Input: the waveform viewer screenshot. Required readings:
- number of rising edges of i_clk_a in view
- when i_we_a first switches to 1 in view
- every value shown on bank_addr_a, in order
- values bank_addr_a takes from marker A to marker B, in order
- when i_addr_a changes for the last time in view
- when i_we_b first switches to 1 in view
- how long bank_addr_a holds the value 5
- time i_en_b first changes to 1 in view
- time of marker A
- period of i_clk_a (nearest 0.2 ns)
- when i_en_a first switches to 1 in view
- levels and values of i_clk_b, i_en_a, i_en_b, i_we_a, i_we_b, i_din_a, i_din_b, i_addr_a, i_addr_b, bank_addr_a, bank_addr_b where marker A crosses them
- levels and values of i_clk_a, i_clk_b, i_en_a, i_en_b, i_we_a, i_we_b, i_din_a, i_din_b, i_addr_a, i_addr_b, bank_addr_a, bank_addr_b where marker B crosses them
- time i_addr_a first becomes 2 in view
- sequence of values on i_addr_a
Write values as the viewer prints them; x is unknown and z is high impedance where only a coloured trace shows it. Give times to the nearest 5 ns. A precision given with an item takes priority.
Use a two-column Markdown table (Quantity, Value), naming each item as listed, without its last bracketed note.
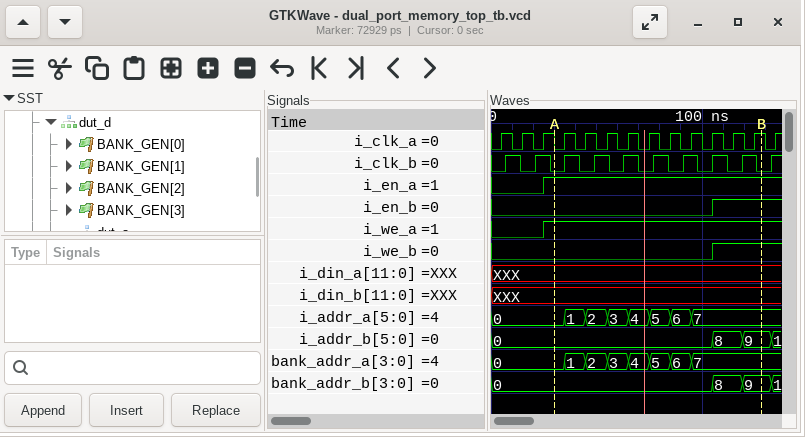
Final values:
| Quantity | Value |
|---|---|
| number of rising edges of i_clk_a in view | 14 |
| when i_we_a first switches to 1 in view | 25 ns |
| every value shown on bank_addr_a, in order | 0, 1, 2, 3, 4, 5, 6, 7 |
| values bank_addr_a takes from marker A to marker B, in order | 0, 1, 2, 3, 4, 5, 6, 7 |
| when i_addr_a changes for the last time in view | 95 ns |
| when i_we_b first switches to 1 in view | 105 ns |
| how long bank_addr_a holds the value 5 | 10 ns |
| time i_en_b first changes to 1 in view | 105 ns |
| time of marker A | 30 ns |
| period of i_clk_a | 10 ns |
| when i_en_a first switches to 1 in view | 25 ns |
| levels and values of i_clk_b, i_en_a, i_en_b, i_we_a, i_we_b, i_din_a, i_din_b, i_addr_a, i_addr_b, bank_addr_a, bank_addr_b where marker A crosses them | i_clk_b=0, i_en_a=1, i_en_b=0, i_we_a=1, i_we_b=0, i_din_a=XXX, i_din_b=XXX, i_addr_a=0, i_addr_b=0, bank_addr_a=0, bank_addr_b=0 |
| levels and values of i_clk_a, i_clk_b, i_en_a, i_en_b, i_we_a, i_we_b, i_din_a, i_din_b, i_addr_a, i_addr_b, bank_addr_a, bank_addr_b where marker B crosses them | i_clk_a=1, i_clk_b=0, i_en_a=1, i_en_b=1, i_we_a=1, i_we_b=1, i_din_a=XXX, i_din_b=XXX, i_addr_a=7, i_addr_b=9, bank_addr_a=7, bank_addr_b=9 |
| time i_addr_a first becomes 2 in view | 45 ns |
| sequence of values on i_addr_a | 0, 1, 2, 3, 4, 5, 6, 7 |
